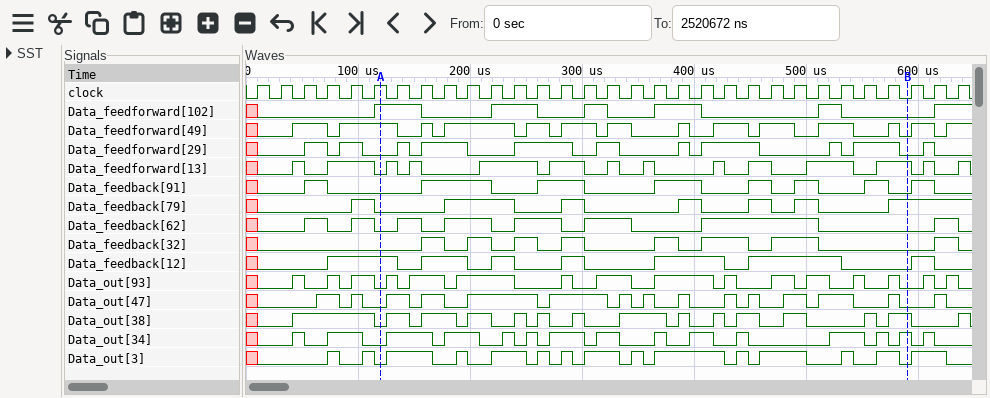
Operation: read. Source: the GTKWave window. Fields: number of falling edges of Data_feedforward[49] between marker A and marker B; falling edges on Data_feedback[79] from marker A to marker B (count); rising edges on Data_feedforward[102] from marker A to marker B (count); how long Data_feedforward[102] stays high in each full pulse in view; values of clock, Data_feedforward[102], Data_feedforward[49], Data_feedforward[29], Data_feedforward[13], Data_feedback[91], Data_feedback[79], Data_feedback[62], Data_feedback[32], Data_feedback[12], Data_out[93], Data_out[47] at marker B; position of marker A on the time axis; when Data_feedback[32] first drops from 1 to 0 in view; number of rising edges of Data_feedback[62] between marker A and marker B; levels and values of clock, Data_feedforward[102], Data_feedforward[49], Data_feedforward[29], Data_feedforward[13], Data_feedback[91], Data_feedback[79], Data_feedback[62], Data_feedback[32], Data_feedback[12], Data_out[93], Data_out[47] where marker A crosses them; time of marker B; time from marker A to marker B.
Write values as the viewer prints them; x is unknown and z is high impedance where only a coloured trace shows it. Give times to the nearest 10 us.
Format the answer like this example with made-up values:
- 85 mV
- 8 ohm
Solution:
- 11
- 5
- 4
- 40 us, 40 us, 20 us, 40 us, 20 us
- clock=0, Data_feedforward[102]=0, Data_feedforward[49]=0, Data_feedforward[29]=0, Data_feedforward[13]=1, Data_feedback[91]=0, Data_feedback[79]=1, Data_feedback[62]=0, Data_feedback[32]=0, Data_feedback[12]=0, Data_out[93]=0, Data_out[47]=0
- 120 us
- 180 us
- 5
- clock=1, Data_feedforward[102]=1, Data_feedforward[49]=1, Data_feedforward[29]=0, Data_feedforward[13]=0, Data_feedback[91]=0, Data_feedback[79]=0, Data_feedback[62]=0, Data_feedback[32]=0, Data_feedback[12]=1, Data_out[93]=0, Data_out[47]=0
- 590 us
- 470 us
